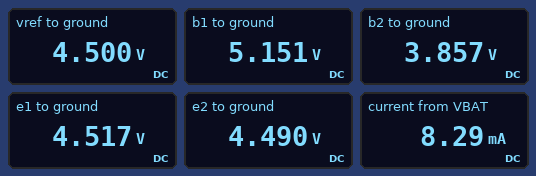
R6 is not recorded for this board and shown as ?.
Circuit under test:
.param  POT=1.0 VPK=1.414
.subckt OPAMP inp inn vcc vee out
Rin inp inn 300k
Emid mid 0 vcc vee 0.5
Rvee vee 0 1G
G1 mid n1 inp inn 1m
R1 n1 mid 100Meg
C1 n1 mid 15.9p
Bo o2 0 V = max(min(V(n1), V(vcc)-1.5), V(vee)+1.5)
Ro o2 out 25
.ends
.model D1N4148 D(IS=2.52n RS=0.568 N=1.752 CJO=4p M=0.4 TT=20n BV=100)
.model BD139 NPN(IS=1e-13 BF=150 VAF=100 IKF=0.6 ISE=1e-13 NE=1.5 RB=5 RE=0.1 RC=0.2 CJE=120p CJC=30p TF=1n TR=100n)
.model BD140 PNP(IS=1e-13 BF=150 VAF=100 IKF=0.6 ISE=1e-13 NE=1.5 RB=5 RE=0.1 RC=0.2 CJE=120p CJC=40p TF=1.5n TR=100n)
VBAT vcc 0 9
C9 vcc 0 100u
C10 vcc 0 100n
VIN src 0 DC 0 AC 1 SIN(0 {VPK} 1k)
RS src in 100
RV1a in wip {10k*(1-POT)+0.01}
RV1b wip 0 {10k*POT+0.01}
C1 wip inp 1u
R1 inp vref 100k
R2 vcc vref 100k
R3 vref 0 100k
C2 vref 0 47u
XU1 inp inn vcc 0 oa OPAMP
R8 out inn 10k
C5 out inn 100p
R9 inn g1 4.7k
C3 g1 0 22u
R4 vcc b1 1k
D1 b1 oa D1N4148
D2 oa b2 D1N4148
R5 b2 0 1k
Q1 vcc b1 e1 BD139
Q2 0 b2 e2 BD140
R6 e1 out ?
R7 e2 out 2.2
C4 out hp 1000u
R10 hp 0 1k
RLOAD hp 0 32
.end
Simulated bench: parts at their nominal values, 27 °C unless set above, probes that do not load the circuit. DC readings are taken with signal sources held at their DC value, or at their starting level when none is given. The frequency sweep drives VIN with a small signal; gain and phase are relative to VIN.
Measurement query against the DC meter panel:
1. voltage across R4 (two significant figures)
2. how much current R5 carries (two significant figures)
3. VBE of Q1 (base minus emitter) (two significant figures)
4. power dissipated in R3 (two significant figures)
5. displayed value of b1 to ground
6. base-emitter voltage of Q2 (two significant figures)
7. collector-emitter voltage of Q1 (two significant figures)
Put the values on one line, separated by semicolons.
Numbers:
3.8 V; 3.9 mA; 630 mV; 200 µW; 5.151 V; -630 mV; 4.5 V
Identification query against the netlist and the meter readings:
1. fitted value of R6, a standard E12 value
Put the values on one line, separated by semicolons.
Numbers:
3.9 Ω
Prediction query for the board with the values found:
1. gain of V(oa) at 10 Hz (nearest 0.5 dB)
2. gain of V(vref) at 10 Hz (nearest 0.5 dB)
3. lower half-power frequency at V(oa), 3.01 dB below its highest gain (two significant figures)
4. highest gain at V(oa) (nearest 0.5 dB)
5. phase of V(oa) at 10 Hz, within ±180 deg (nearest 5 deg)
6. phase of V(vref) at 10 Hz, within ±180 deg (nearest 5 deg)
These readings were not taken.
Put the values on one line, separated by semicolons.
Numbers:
10.5 dB; -49.5 dB; 2.9 Hz; 11.0 dB; 20 deg; -80 deg
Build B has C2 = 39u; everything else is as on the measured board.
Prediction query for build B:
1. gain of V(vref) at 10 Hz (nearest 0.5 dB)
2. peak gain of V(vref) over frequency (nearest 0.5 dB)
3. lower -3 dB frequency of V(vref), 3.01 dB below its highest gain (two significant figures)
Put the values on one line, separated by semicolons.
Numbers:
-48.0 dB; -32.5 dB; 73 mHz
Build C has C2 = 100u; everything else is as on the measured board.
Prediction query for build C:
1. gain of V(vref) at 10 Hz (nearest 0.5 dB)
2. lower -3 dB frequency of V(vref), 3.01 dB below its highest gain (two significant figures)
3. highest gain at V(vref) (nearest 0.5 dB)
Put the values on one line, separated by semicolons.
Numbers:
-56.0 dB; 30 mHz; -40.5 dB
